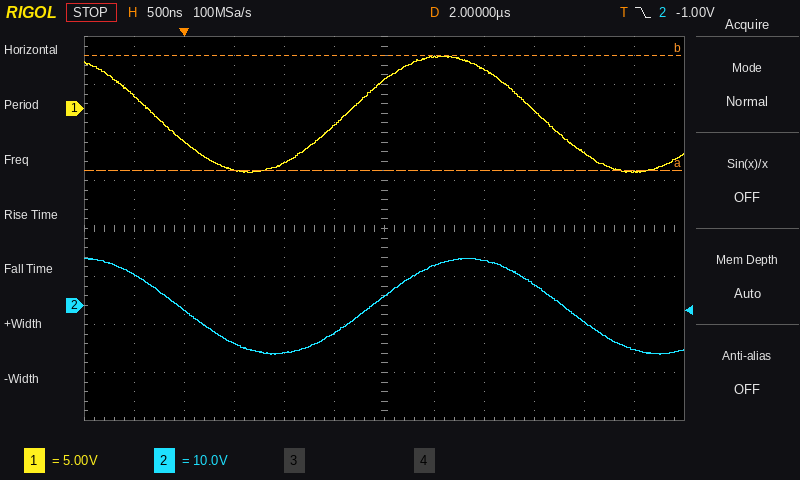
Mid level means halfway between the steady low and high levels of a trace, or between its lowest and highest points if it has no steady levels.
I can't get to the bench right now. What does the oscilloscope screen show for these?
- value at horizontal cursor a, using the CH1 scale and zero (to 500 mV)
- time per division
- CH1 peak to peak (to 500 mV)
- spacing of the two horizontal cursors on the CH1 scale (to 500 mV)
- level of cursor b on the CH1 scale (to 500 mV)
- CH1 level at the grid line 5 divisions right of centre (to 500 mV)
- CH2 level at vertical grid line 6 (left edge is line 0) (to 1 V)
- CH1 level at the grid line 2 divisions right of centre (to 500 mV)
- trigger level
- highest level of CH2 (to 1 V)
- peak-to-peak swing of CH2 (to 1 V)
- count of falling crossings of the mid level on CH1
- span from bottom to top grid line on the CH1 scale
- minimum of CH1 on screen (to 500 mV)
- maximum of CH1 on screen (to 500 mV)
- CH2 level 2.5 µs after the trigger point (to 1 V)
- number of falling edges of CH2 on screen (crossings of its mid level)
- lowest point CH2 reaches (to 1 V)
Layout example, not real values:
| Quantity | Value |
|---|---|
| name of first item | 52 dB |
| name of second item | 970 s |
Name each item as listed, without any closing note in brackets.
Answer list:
| Quantity | Value |
|---|---|
| value at horizontal cursor a, using the CH1 scale and zero | -6.5 V |
| time per division | 500 ns |
| CH1 peak to peak | 12.0 V |
| spacing of the two horizontal cursors on the CH1 scale | 12.0 V |
| level of cursor b on the CH1 scale | 5.5 V |
| CH1 level at the grid line 5 divisions right of centre | -6.5 V |
| CH2 level at vertical grid line 6 (left edge is line 0) | 2 V |
| CH1 level at the grid line 2 divisions right of centre | 4.0 V |
| trigger level | -1.00 V |
| highest level of CH2 | 10 V |
| peak-to-peak swing of CH2 | 20 V |
| count of falling crossings of the mid level on CH1 | 2 |
| span from bottom to top grid line on the CH1 scale | 40 V |
| minimum of CH1 on screen | -6.5 V |
| maximum of CH1 on screen | 5.5 V |
| CH2 level 2.5 µs after the trigger point | 8 V |
| number of falling edges of CH2 on screen | 2 |
| lowest point CH2 reaches | -10 V |
